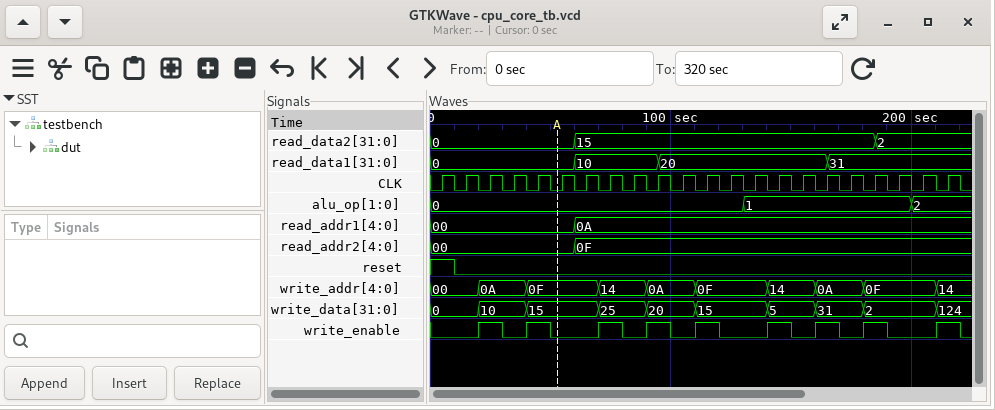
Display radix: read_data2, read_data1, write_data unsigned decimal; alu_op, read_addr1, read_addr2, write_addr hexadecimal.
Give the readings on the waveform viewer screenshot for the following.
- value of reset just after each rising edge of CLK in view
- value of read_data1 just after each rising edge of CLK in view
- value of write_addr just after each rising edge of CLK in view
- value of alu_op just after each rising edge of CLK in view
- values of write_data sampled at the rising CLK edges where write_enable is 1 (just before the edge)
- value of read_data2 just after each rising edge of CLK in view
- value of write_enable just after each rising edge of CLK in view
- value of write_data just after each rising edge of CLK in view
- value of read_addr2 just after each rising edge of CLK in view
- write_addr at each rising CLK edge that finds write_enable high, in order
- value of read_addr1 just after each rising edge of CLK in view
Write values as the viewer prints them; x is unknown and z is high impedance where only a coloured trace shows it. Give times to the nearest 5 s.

1 0 0 0 0 0 0 0 0 0 0 0 0 0 0 0 0 0 0 0 0 0
0, 0, 0, 0, 0, 0, 10, 10, 10, 20, 20, 20, 20, 20, 20, 20, 31, 31, 31, 31, 31, 31
00, 00, 0A, 0A, 0F, 0F, 0F, 14, 14, 0A, 0A, 0F, 0F, 0F, 14, 14, 0A, 0A, 0F, 0F, 0F, 14
0, 0, 0, 0, 0, 0, 0, 0, 0, 0, 0, 0, 0, 1, 1, 1, 1, 1, 1, 1, 2, 2
10, 15, 25, 20, 15, 5, 31, 2, 124
0, 0, 0, 0, 0, 0, 15, 15, 15, 15, 15, 15, 15, 15, 15, 15, 15, 15, 2, 2, 2, 2
0 0 1 0 1 0 0 1 0 1 0 1 0 0 1 0 1 0 1 0 0 1
0, 0, 10, 10, 15, 15, 15, 25, 25, 20, 20, 15, 15, 15, 5, 5, 31, 31, 2, 2, 2, 124
00, 00, 00, 00, 00, 00, 0F, 0F, 0F, 0F, 0F, 0F, 0F, 0F, 0F, 0F, 0F, 0F, 0F, 0F, 0F, 0F
0A, 0F, 14, 0A, 0F, 14, 0A, 0F, 14
00, 00, 00, 00, 00, 00, 0A, 0A, 0A, 0A, 0A, 0A, 0A, 0A, 0A, 0A, 0A, 0A, 0A, 0A, 0A, 0A
